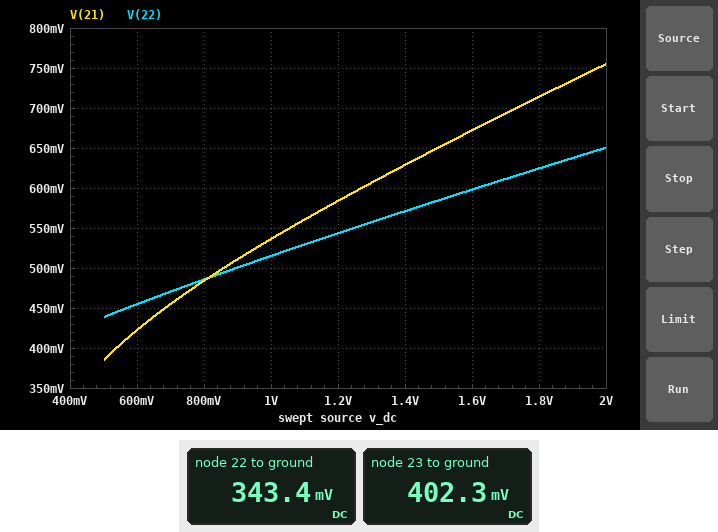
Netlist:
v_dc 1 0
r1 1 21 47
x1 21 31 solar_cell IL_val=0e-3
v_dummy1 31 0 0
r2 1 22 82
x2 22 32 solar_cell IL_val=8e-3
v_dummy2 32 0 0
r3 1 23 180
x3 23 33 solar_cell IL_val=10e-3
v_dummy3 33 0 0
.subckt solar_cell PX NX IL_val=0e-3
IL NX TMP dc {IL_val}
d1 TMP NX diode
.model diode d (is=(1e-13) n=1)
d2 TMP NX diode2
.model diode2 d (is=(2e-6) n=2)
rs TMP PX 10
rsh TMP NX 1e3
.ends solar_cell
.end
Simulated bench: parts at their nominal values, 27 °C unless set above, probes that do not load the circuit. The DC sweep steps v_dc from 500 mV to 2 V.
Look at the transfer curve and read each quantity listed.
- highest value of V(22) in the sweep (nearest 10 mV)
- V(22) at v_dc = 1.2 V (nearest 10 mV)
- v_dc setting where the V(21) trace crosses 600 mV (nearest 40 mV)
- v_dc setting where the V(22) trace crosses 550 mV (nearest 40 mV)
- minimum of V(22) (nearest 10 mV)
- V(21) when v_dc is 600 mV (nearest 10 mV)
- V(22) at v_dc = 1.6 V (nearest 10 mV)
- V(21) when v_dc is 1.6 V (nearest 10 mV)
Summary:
650 mV
540 mV
1.28 V
1.24 V
440 mV
420 mV
600 mV
670 mV
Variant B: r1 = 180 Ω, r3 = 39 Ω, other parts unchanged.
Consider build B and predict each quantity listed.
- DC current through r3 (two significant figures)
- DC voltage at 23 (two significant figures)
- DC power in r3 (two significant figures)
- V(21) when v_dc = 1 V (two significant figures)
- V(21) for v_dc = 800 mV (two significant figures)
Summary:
7.4 mA
290 mV
2.1 mW
410 mV
380 mV
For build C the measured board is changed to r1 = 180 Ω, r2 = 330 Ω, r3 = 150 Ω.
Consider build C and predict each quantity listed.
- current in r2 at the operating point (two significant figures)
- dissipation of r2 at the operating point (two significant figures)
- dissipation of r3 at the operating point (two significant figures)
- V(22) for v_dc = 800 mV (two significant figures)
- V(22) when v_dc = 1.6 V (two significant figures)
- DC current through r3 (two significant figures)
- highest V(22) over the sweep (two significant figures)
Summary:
1.2 mA
500 µW
1.0 mW
440 mV
480 mV
2.6 mA
500 mV
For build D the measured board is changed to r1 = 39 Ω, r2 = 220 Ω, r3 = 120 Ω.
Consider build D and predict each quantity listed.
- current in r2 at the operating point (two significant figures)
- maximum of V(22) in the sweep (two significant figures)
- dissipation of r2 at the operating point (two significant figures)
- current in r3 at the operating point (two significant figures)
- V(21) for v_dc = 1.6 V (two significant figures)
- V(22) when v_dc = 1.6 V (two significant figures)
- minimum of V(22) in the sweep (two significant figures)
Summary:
1.8 mA
530 mV
710 µW
3.2 mA
710 mV
500 mV
430 mV
